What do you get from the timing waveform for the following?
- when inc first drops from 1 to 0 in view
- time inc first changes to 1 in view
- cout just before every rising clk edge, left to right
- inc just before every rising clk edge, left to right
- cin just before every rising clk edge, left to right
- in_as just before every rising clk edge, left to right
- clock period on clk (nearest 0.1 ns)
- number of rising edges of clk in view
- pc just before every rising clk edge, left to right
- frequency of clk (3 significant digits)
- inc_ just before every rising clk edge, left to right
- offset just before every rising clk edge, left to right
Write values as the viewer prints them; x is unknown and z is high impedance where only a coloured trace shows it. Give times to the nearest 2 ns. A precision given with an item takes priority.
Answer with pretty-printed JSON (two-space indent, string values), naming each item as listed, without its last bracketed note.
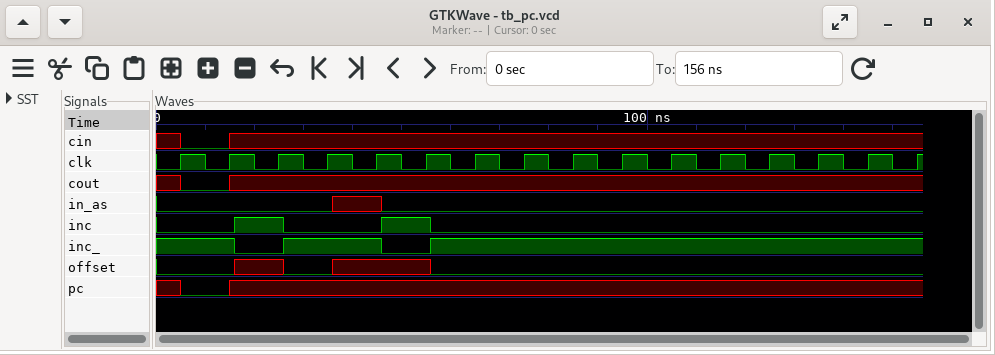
{
  "when inc first drops from 1 to 0 in view": "26 ns",
  "time inc first changes to 1 in view": "16 ns",
  "cout just before every rising clk edge, left to right": "x 0 x x x x x x x x x x x x x x",
  "inc just before every rising clk edge, left to right": "0 0 1 0 0 1 0 0 0 0 0 0 0 0 0 0",
  "cin just before every rising clk edge, left to right": "x 0 x x x x x x x x x x x x x x",
  "in_as just before every rising clk edge, left to right": "0 0 0 0 x 0 0 0 0 0 0 0 0 0 0 0",
  "clock period on clk": "10 ns",
  "number of rising edges of clk in view": "16",
  "pc just before every rising clk edge, left to right": "x 0 x x x x x x x x x x x x x x",
  "frequency of clk": "100 MHz",
  "inc_ just before every rising clk edge, left to right": "1 1 0 1 1 0 1 1 1 1 1 1 1 1 1 1",
  "offset just before every rising clk edge, left to right": "0 0 x 0 x x 0 0 0 0 0 0 0 0 0 0"
}
